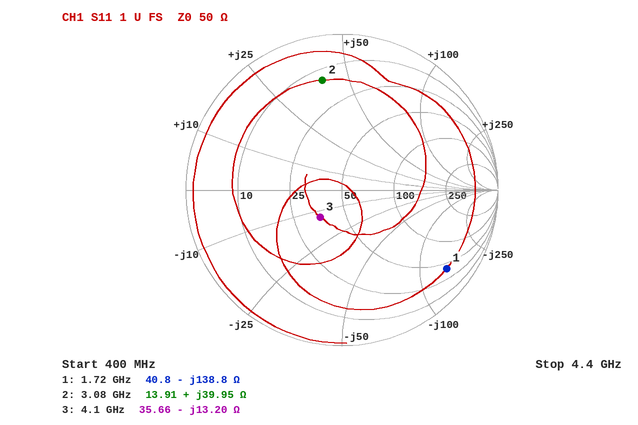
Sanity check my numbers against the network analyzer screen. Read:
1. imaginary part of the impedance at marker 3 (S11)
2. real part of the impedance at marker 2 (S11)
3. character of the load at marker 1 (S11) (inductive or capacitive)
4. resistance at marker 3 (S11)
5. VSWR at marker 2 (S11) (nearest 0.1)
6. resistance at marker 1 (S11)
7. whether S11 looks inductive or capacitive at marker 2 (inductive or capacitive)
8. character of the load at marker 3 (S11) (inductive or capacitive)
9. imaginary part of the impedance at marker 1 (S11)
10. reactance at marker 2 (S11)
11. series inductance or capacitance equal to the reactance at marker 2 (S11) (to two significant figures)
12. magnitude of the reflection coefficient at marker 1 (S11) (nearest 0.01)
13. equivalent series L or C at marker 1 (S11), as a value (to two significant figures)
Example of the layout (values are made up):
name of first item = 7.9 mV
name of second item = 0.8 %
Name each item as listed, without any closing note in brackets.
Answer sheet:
imaginary part of the impedance at marker 3 = -13.20 Ω
real part of the impedance at marker 2 = 13.91 Ω
character of the load at marker 1 (S11) = capacitive
resistance at marker 3 = 35.66 Ω
VSWR at marker 2 (S11) = 6.0
resistance at marker 1 = 40.8 Ω
whether S11 looks inductive or capacitive at marker 2 = inductive
character of the load at marker 3 (S11) = capacitive
imaginary part of the impedance at marker 1 = -138.8 Ω
reactance at marker 2 = +39.95 Ω
series inductance or capacitance equal to the reactance at marker 2 (S11) = 2.1 nH
magnitude of the reflection coefficient at marker 1 (S11) = 0.84
equivalent series L or C at marker 1 (S11), as a value = 670 fF
